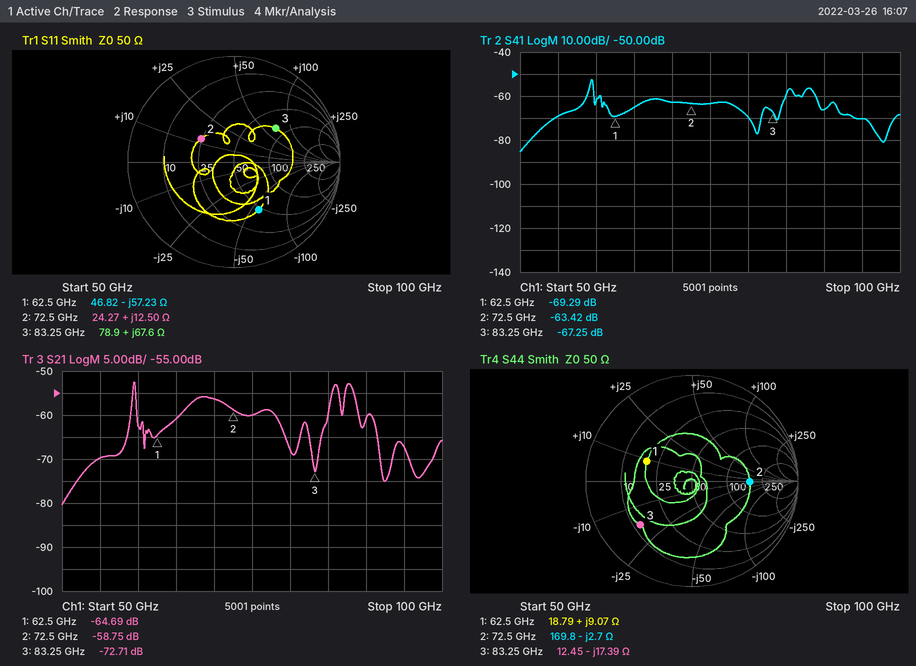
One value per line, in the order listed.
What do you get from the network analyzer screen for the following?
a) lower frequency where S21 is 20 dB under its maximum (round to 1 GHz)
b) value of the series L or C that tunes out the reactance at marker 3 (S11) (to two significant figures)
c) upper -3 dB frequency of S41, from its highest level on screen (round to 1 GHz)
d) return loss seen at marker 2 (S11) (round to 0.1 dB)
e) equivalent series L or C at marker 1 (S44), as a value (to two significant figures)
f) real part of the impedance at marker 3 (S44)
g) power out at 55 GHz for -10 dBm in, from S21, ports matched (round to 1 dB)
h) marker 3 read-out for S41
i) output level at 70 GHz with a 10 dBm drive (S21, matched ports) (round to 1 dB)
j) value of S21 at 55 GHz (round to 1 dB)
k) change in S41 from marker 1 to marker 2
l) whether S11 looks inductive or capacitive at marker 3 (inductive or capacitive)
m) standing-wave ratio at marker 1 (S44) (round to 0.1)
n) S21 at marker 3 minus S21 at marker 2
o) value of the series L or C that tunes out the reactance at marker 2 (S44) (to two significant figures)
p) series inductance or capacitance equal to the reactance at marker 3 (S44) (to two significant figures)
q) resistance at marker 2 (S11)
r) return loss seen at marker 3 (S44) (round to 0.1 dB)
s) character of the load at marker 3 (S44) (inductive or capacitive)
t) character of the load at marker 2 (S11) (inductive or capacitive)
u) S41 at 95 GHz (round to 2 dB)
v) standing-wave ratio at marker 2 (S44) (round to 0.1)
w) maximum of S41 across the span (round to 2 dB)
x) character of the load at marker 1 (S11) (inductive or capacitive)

53 GHz
28 fF
60 GHz
8.4 dB
23 pH
12.45 Ω
-80 dBm
-67.25 dB
-46 dBm
-70 dB
5.87 dB
inductive
2.8
-13.96 dB
5.9 pH
110 fF
24.27 Ω
3.9 dB
capacitive
inductive
-70 dB
3.4
-52 dB
capacitive
